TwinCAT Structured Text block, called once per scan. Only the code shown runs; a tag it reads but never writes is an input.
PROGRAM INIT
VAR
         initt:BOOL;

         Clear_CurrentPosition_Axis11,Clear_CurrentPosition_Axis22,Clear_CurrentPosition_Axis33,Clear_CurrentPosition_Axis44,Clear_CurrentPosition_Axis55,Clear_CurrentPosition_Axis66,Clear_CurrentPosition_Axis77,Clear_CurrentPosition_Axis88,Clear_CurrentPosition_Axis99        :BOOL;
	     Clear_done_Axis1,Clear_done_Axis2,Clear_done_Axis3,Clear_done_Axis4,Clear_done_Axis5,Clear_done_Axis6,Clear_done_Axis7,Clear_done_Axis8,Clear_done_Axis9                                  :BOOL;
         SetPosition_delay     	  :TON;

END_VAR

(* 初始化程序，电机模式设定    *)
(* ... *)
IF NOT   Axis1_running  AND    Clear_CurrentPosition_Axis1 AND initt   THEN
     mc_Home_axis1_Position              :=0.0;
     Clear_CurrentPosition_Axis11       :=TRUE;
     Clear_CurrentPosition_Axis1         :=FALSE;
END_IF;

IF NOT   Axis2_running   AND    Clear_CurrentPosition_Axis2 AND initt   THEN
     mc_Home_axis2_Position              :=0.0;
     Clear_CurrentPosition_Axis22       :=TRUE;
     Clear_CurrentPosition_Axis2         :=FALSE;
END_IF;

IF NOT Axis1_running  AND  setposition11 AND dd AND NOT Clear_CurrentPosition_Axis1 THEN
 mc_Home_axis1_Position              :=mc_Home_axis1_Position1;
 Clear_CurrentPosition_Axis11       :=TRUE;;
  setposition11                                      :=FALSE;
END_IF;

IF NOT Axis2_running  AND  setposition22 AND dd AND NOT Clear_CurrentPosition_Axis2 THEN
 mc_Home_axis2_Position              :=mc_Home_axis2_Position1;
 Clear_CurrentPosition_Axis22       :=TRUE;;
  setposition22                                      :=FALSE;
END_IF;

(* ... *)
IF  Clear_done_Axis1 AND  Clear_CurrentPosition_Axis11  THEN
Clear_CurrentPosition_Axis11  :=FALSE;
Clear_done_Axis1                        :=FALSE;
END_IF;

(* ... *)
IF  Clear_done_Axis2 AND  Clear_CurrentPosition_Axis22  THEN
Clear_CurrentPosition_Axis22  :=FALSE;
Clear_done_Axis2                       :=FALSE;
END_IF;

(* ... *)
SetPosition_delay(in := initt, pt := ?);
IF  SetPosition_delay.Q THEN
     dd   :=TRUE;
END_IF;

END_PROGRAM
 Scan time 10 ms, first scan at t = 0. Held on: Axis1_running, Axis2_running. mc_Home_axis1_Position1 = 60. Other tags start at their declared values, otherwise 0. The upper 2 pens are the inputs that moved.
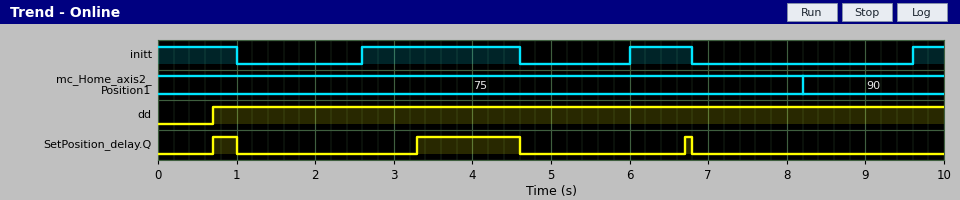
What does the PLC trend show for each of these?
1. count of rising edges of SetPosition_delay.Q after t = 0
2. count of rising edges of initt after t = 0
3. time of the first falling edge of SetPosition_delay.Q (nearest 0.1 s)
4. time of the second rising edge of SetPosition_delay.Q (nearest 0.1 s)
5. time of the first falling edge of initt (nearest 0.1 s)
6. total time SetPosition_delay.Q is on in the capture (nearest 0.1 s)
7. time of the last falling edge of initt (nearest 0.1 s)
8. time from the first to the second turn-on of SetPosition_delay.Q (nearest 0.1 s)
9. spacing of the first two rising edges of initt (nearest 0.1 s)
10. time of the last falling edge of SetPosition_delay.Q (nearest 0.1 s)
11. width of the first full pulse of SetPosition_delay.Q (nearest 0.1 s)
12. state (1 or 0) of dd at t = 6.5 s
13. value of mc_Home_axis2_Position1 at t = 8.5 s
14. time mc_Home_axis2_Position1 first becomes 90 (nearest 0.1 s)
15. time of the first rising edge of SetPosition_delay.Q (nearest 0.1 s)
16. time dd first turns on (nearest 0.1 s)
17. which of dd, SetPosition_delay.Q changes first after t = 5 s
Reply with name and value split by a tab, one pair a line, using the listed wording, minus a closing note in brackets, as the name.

count of rising edges of SetPosition_delay.Q after t = 0	3
count of rising edges of initt after t = 0	3
time of the first falling edge of SetPosition_delay.Q	1.0 s
time of the second rising edge of SetPosition_delay.Q	3.3 s
time of the first falling edge of initt	1.0 s
total time SetPosition_delay.Q is on in the capture	1.7 s
time of the last falling edge of initt	6.8 s
time from the first to the second turn-on of SetPosition_delay.Q	2.6 s
spacing of the first two rising edges of initt	3.4 s
time of the last falling edge of SetPosition_delay.Q	6.8 s
width of the first full pulse of SetPosition_delay.Q	0.3 s
state (1 or 0) of dd at t = 6.5 s	1
value of mc_Home_axis2_Position1 at t = 8.5 s	90
time mc_Home_axis2_Position1 first becomes 90	8.2 s
time of the first rising edge of SetPosition_delay.Q	0.7 s
time dd first turns on	0.7 s
which of dd, SetPosition_delay.Q changes first after t = 5 s	SetPosition_delay.Q
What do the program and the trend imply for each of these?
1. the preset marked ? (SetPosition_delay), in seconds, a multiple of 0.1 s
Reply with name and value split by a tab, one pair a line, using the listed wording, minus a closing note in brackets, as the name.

the preset marked ? (SetPosition_delay), in seconds, a multiple of 0.1 s	0.7 s
